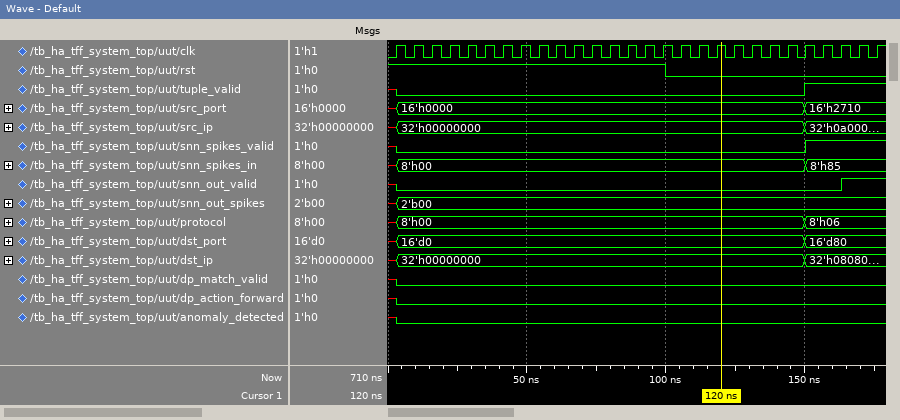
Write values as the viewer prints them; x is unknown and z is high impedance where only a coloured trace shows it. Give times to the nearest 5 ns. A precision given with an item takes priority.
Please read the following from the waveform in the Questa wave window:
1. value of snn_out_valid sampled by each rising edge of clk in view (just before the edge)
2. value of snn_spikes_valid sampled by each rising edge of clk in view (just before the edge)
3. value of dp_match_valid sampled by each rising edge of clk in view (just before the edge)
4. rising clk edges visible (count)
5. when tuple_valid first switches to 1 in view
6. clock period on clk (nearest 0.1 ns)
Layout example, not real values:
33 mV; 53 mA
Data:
x 0 0 0 0 0 0 0 0 0 0 0 0 0 0 0 0 0 0 0 0 0 0 0 0 0 1 1; x 0 0 0 0 0 0 0 0 0 0 0 0 0 0 0 0 0 0 0 0 0 0 0 1 1 1 1; x 0 0 0 0 0 0 0 0 0 0 0 0 0 0 0 0 0 0 0 0 0 0 0 0 0 0 0; 28; 150 ns; 6.4 ns
